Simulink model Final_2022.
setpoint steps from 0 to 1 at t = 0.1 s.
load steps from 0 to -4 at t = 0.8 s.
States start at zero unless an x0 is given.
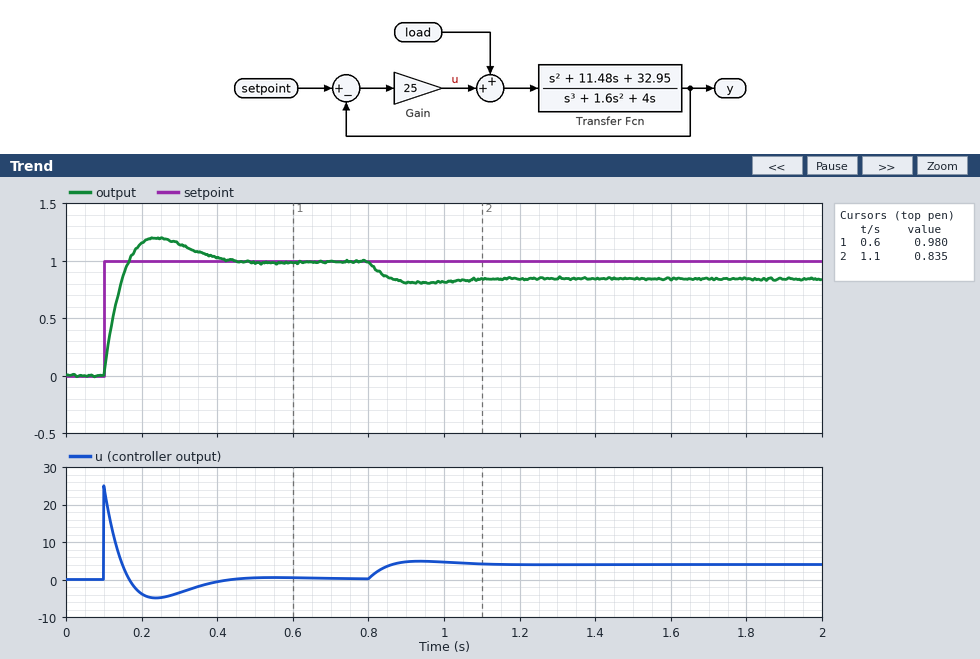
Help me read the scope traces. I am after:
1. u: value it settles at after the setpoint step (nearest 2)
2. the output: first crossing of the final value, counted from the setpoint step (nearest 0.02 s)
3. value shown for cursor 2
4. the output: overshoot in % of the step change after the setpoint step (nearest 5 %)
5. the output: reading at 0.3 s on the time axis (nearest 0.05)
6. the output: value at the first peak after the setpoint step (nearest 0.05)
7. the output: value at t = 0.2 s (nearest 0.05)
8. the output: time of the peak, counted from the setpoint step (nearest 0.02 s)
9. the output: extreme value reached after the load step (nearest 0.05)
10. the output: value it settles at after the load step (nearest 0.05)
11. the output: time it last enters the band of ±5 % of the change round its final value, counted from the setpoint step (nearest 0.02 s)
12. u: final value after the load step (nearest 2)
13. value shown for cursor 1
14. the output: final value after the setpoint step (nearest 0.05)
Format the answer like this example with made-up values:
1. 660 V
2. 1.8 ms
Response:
1. 0
2. 0.06 s
3. 0.835
4. 20 %
5. 1.15
6. 1.20
7. 1.15
8. 0.14 s
9. 0.80
10. 0.85
11. 0.28 s
12. 4
13. 0.980
14. 1.00
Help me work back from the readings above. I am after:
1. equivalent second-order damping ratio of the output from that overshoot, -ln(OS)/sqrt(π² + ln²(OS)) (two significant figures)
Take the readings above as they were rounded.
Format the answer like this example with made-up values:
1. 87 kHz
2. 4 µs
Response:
1. 0.46
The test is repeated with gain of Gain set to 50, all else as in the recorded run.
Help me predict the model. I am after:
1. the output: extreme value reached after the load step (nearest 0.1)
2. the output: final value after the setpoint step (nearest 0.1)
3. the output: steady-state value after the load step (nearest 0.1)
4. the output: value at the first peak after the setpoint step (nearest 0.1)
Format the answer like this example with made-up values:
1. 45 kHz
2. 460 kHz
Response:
1. 0.9
2. 1.0
3. 0.9
4. 1.1
